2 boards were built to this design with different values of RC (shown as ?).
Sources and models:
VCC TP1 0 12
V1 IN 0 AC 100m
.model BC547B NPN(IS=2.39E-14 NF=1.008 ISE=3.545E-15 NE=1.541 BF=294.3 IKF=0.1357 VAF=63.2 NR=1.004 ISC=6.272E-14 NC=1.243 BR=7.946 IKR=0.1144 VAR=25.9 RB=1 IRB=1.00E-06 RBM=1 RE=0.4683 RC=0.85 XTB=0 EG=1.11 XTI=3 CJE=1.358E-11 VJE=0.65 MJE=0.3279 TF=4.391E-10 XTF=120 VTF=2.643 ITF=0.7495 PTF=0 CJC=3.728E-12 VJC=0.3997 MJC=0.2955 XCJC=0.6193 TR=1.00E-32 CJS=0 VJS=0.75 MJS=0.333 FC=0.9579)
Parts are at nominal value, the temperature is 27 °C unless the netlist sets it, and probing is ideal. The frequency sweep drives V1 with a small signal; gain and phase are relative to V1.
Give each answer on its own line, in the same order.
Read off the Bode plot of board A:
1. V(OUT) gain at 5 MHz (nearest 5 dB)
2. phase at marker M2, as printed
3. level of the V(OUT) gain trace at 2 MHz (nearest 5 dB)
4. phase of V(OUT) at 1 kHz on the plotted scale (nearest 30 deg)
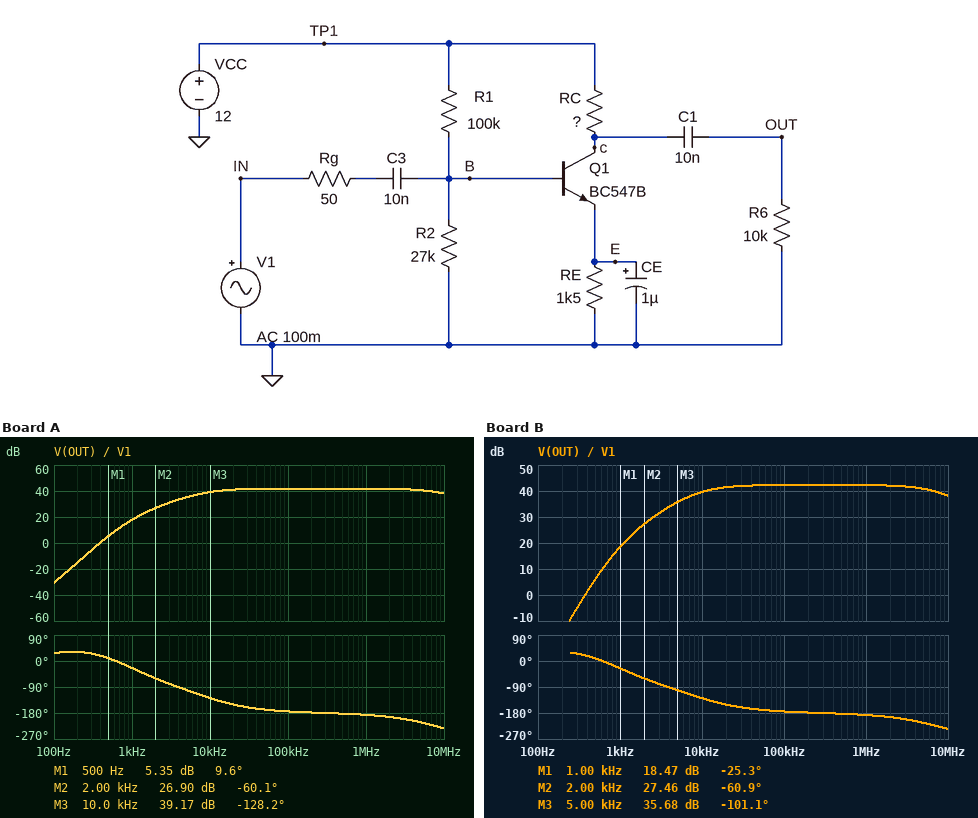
40 dB
-60.1 deg
40 dB
-30 deg
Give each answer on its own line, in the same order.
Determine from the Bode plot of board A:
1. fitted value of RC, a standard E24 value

4.3 kΩ
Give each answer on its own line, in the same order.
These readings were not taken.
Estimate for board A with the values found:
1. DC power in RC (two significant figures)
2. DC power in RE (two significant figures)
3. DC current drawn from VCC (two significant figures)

6.3 mW
2.2 mW
1.3 mA
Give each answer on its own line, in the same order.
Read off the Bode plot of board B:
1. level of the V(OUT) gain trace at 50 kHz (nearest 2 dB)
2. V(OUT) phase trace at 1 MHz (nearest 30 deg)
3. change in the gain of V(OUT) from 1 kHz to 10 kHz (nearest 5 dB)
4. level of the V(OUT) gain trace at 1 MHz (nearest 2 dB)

42 dB
-180 deg
20 dB
42 dB
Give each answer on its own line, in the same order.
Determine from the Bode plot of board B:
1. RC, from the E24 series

4.7 kΩ
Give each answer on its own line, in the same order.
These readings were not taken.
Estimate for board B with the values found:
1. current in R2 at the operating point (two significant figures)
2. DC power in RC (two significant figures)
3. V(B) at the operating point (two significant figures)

91 µA
6.9 mW
2.5 V
